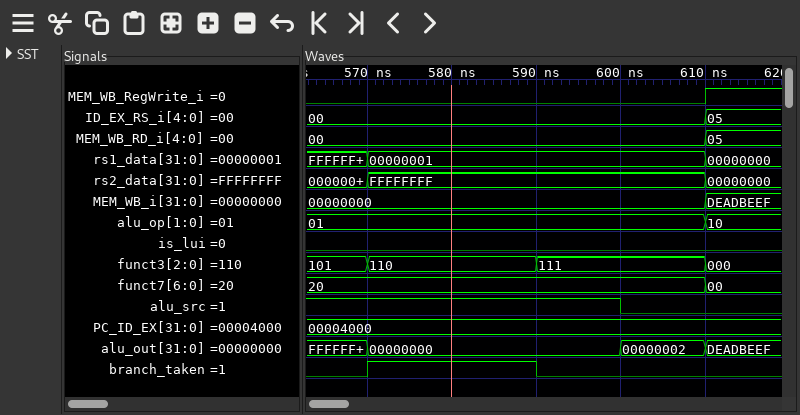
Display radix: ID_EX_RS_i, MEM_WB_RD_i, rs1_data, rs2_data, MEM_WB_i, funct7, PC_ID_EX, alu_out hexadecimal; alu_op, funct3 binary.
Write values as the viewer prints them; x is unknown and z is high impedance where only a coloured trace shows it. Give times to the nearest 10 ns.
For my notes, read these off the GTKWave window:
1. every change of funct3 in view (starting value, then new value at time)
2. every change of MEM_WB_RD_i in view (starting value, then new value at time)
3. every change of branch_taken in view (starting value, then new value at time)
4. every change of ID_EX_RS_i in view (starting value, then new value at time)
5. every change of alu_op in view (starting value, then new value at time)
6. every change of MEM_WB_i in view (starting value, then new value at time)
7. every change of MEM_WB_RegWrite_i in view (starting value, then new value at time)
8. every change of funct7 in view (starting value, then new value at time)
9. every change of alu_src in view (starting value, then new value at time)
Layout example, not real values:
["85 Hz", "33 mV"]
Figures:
["101, 110 at 570 ns, 111 at 590 ns, 000 at 610 ns", "00, 05 at 610 ns", "0, 1 at 570 ns, 0 at 590 ns", "00, 05 at 610 ns", "01, 10 at 610 ns", "00000000, DEADBEEF at 610 ns", "0, 1 at 610 ns", "20, 00 at 610 ns", "1, 0 at 600 ns"]
